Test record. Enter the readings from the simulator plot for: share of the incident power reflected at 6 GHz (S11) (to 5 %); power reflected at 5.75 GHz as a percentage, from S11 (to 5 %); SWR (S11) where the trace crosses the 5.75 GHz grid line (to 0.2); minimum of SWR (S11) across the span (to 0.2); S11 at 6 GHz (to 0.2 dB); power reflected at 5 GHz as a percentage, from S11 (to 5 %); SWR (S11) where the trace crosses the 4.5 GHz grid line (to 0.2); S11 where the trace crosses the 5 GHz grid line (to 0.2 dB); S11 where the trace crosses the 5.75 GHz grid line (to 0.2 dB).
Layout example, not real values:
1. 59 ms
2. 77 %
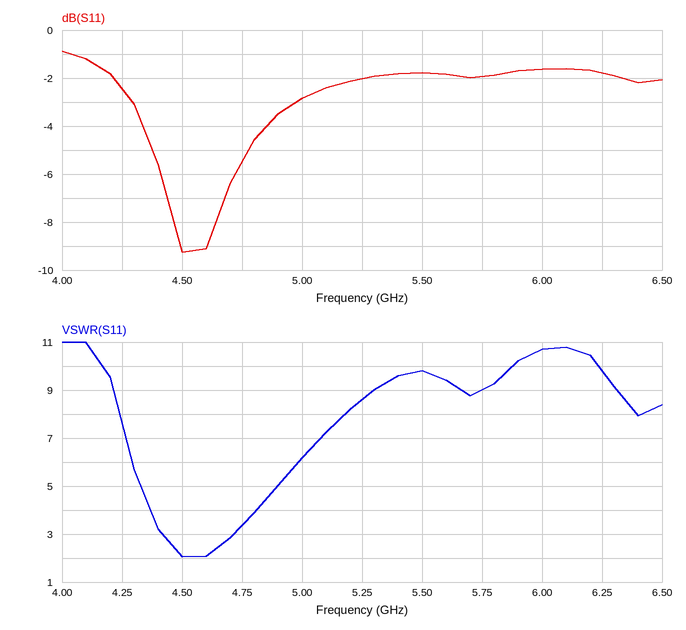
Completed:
1. 70 %
2. 65 %
3. 9.0
4. 2.0
5. -1.6 dB
6. 50 %
7. 2.0
8. -2.8 dB
9. -2.0 dB
